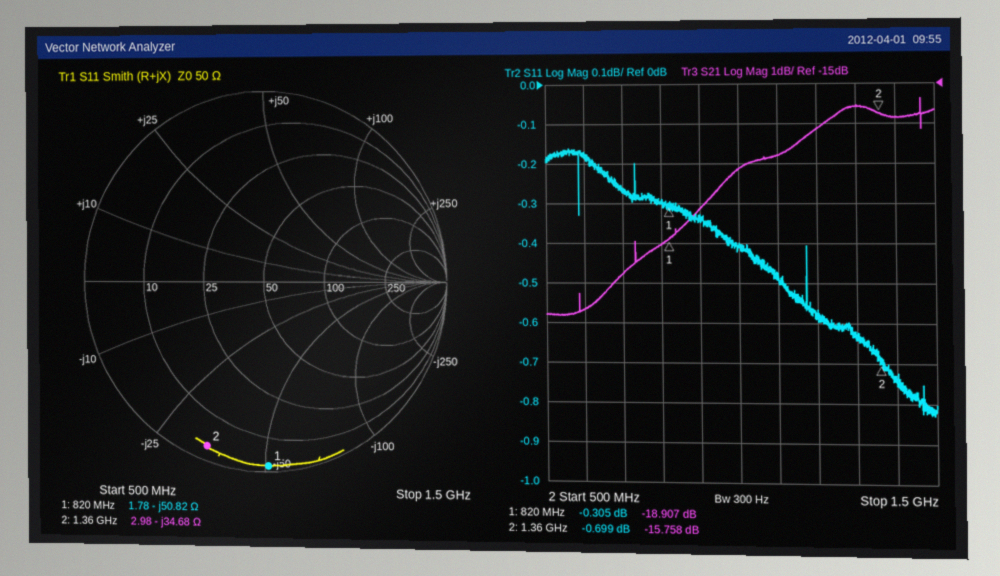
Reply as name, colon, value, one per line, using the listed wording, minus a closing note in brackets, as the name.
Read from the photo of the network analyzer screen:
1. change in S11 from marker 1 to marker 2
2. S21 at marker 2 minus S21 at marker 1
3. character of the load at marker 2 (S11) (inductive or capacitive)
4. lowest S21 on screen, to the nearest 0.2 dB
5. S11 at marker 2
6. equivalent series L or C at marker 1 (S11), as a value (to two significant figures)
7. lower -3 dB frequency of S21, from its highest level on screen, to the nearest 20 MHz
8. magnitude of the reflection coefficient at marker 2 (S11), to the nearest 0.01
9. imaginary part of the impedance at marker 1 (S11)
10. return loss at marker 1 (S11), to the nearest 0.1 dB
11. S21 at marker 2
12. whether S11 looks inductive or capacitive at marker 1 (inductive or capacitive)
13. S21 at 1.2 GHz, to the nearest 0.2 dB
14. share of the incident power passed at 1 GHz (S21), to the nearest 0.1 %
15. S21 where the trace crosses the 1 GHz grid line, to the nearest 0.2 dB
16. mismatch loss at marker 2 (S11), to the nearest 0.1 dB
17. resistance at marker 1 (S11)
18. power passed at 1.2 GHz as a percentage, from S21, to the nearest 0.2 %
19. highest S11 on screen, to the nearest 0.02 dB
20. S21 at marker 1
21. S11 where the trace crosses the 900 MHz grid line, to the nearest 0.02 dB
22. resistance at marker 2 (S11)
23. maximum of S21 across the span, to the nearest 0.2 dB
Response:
change in S11 from marker 1 to marker 2: -0.394 dB
S21 at marker 2 minus S21 at marker 1: 3.149 dB
character of the load at marker 2 (S11): capacitive
lowest S21 on screen, to the nearest 0.2 dB: -20.8 dB
S11 at marker 2: -0.699 dB
equivalent series L or C at marker 1 (S11), as a value: 3.8 pF
lower -3 dB frequency of S21, from its highest level on screen, to the nearest 20 MHz: 880 MHz
magnitude of the reflection coefficient at marker 2 (S11), to the nearest 0.01: 0.92
imaginary part of the impedance at marker 1: -50.82 Ω
return loss at marker 1 (S11), to the nearest 0.1 dB: 0.3 dB
S21 at marker 2: -15.758 dB
whether S11 looks inductive or capacitive at marker 1: capacitive
S21 at 1.2 GHz, to the nearest 0.2 dB: -16.2 dB
share of the incident power passed at 1 GHz (S21), to the nearest 0.1 %: 1.9 %
S21 where the trace crosses the 1 GHz grid line, to the nearest 0.2 dB: -17.2 dB
mismatch loss at marker 2 (S11), to the nearest 0.1 dB: 8.3 dB
resistance at marker 1: 1.78 Ω
power passed at 1.2 GHz as a percentage, from S21, to the nearest 0.2 %: 2.4 %
highest S11 on screen, to the nearest 0.02 dB: -0.16 dB
S21 at marker 1: -18.907 dB
S11 where the trace crosses the 900 MHz grid line, to the nearest 0.02 dB: -0.34 dB
resistance at marker 2: 2.98 Ω
maximum of S21 across the span, to the nearest 0.2 dB: -15.4 dB
